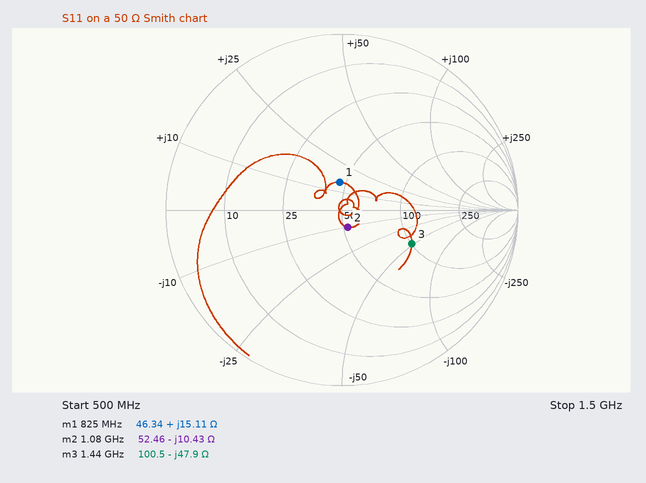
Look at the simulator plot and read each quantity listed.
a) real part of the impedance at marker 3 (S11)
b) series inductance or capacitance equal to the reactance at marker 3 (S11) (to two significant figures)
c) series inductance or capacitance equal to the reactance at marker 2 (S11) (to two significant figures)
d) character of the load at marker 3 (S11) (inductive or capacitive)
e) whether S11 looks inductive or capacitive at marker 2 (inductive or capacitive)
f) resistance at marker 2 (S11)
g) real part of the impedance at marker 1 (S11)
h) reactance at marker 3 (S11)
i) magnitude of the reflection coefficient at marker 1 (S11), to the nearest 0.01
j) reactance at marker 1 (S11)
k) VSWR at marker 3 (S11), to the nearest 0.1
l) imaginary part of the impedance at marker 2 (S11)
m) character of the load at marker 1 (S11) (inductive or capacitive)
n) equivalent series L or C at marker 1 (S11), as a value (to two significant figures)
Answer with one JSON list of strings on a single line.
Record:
["100.5 Ω", "2.3 pF", "14 pF", "capacitive", "capacitive", "52.46 Ω", "46.34 Ω", "-47.9 Ω", "0.16", "+15.11 Ω", "2.6", "-10.43 Ω", "inductive", "2.9 nH"]
